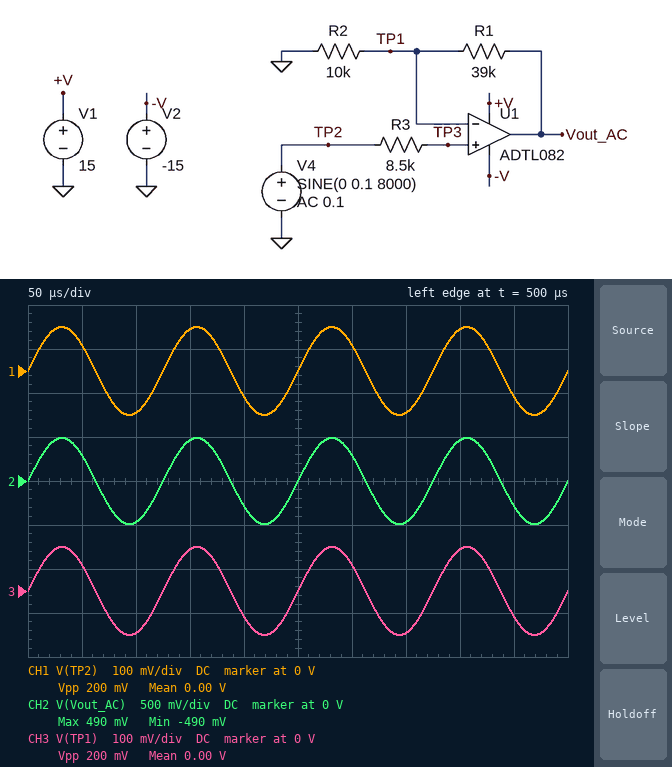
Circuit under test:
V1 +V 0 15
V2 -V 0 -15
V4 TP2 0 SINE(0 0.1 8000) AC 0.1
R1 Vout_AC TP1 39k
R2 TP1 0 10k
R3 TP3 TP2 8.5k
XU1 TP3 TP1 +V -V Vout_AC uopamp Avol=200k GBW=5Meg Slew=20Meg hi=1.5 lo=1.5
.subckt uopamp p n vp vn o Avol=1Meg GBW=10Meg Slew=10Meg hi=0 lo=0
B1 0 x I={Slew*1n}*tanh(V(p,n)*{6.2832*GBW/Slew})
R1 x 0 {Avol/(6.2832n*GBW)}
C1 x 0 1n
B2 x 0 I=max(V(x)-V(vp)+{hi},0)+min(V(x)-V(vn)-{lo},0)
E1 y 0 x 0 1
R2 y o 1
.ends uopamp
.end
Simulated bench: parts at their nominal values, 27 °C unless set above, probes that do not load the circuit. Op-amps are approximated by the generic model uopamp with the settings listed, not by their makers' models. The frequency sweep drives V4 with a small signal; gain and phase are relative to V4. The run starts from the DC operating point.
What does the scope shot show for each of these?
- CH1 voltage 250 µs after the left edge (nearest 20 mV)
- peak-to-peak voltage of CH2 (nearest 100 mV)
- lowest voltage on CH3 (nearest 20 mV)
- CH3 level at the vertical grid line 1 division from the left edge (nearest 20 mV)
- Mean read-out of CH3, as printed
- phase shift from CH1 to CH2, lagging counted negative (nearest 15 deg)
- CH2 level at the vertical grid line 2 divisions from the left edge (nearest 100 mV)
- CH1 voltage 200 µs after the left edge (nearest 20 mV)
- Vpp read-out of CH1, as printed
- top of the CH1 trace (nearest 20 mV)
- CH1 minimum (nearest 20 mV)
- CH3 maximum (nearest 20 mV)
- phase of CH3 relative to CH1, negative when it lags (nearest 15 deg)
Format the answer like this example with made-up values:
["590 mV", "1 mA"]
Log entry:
["0 V", "1.0 V", "-100 mV", "60 mV", "0.00 V", "0 deg", "-500 mV", "-60 mV", "200 mV", "100 mV", "-100 mV", "100 mV", "0 deg"]
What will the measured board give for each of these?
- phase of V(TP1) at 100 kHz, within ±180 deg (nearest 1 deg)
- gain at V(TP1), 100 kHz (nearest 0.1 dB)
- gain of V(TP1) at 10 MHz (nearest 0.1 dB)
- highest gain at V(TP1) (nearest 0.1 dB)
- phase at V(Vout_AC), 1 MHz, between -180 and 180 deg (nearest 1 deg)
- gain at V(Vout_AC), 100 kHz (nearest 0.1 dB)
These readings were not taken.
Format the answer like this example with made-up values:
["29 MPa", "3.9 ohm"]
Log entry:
["-6 deg", "0 dB", "-19.9 dB", "0 dB", "-44 deg", "13.8 dB"]
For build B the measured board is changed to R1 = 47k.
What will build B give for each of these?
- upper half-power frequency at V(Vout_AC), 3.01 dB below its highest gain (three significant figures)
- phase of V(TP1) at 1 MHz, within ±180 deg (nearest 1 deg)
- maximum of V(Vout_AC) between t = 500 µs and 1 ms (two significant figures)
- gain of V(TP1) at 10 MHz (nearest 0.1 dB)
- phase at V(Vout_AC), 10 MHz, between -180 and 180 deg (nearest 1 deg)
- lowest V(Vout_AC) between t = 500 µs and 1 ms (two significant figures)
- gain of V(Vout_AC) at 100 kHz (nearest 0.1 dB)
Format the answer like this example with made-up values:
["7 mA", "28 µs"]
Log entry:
["877 kHz", "-49 deg", "570 mV", "-21.2 dB", "-85 deg", "-570 mV", "15.1 dB"]
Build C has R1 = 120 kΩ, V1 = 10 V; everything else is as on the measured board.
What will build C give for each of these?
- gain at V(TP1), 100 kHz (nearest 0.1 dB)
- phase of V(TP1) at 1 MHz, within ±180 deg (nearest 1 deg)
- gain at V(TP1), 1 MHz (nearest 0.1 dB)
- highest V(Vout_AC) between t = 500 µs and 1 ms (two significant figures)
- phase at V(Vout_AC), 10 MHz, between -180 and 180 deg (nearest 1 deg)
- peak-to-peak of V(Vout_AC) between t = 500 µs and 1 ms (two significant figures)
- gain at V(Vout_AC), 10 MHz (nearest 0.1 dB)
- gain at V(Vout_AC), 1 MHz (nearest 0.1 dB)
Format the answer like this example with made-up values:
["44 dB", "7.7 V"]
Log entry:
["-0.3 dB", "-69 deg", "-8.9 dB", "1.3 V", "-88 deg", "2.6 V", "-6.0 dB", "13.4 dB"]
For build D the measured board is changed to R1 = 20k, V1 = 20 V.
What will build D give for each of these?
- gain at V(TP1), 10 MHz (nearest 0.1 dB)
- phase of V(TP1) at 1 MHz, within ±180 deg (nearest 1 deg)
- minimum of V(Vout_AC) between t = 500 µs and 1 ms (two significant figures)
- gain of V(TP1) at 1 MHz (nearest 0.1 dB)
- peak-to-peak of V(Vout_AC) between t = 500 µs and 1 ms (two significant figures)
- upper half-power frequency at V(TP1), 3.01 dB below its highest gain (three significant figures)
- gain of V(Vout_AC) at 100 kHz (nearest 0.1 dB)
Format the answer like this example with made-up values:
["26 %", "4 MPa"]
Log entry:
["-15.7 dB", "-31 deg", "-300 mV", "-1.3 dB", "600 mV", "1.67 MHz", "9.5 dB"]
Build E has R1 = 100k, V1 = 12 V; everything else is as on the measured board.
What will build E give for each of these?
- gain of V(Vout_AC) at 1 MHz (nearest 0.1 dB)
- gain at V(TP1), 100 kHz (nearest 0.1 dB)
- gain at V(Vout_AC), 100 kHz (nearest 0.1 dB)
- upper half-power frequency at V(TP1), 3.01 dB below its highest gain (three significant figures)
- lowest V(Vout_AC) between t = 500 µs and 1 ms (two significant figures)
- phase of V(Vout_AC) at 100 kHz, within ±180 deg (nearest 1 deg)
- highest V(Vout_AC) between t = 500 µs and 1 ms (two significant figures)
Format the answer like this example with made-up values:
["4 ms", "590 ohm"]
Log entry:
["13.2 dB", "-0.2 dB", "20.6 dB", "455 kHz", "-1.1 V", "-12 deg", "1.1 V"]
